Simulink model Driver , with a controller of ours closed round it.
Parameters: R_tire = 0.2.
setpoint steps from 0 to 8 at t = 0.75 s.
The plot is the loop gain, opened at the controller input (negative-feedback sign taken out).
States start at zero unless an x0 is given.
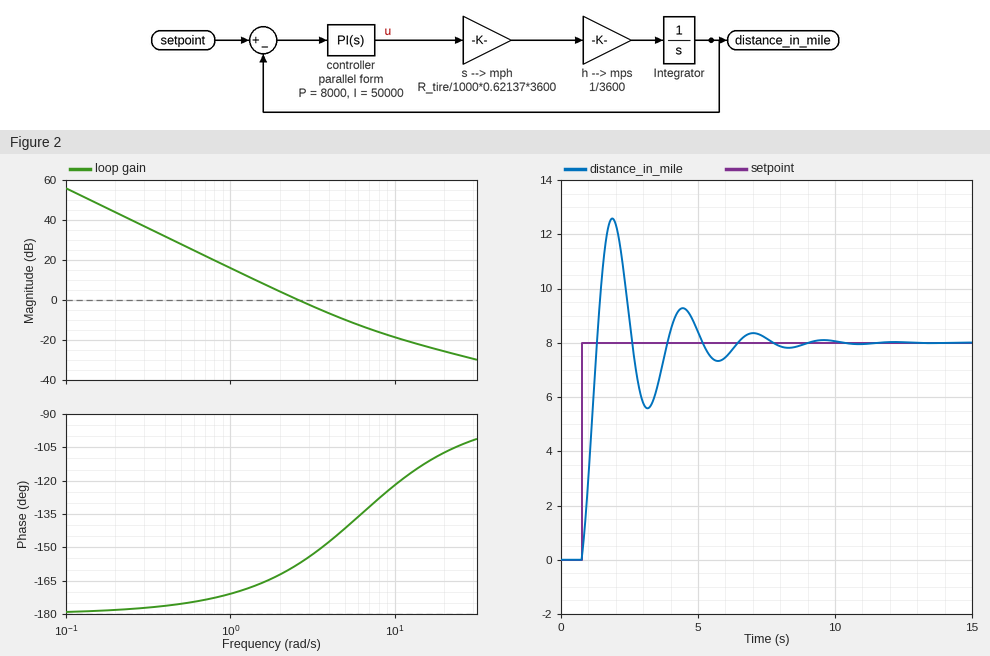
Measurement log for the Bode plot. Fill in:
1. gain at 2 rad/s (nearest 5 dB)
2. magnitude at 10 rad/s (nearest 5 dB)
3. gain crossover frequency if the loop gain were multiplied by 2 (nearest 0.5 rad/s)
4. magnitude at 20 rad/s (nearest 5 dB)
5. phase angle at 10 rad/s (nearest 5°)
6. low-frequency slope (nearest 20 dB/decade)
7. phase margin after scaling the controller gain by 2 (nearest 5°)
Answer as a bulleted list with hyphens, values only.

- 5 dB
- -20 dB
- 4.0 rad/s
- -25 dB
- -120°
- -40 dB/decade
- 30°
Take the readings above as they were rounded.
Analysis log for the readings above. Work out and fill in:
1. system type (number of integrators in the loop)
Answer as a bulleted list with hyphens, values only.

- 2
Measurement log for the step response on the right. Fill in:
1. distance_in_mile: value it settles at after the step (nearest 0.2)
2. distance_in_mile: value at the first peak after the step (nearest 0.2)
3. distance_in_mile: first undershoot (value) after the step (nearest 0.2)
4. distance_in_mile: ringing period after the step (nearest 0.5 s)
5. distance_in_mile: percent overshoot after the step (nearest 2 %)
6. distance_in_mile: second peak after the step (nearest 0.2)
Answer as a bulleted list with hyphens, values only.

- 8.0
- 12.6
- 5.6
- 2.5 s
- 58 %
- 9.2
